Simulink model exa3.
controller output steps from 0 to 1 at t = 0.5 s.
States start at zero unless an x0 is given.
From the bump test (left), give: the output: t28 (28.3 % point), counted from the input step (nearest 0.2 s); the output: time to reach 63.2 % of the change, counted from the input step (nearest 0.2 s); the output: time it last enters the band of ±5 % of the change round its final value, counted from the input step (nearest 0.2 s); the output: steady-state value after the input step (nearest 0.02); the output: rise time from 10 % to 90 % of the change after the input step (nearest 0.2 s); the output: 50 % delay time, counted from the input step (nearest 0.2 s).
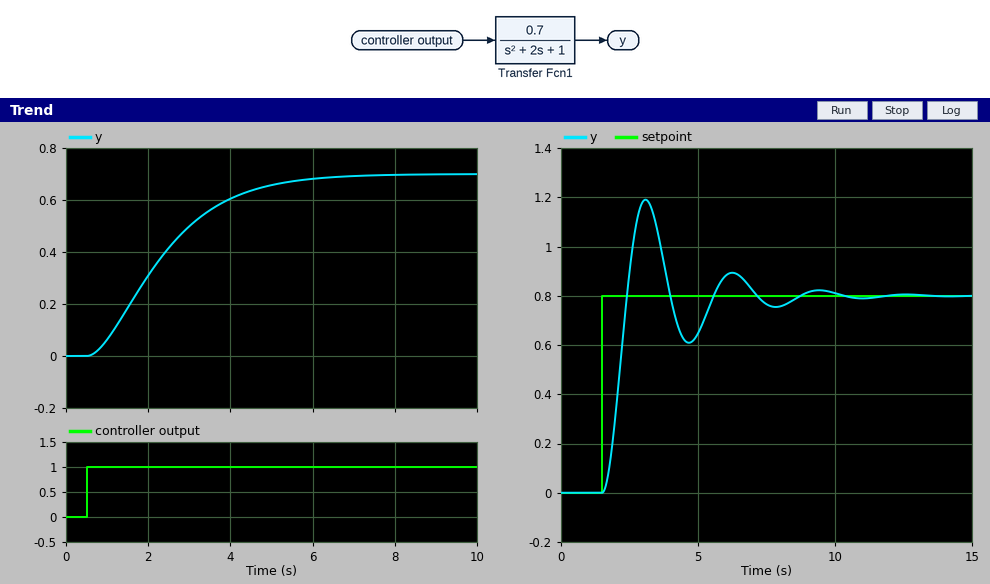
1.0 s
2.2 s
4.8 s
0.70
3.4 s
1.6 s
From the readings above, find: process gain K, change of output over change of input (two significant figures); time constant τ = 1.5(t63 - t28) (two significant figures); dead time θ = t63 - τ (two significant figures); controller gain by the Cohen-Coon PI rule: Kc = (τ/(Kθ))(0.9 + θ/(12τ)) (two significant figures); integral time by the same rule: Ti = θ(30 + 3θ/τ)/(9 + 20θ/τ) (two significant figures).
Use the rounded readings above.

0.70
1.8 s
0.40 s
5.9
0.91 s
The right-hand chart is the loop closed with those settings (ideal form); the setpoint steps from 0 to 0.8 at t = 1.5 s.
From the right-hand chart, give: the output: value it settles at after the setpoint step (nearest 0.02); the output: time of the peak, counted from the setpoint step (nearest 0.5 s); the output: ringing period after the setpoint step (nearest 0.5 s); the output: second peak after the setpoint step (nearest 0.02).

0.80
1.5 s
3.0 s
0.90
